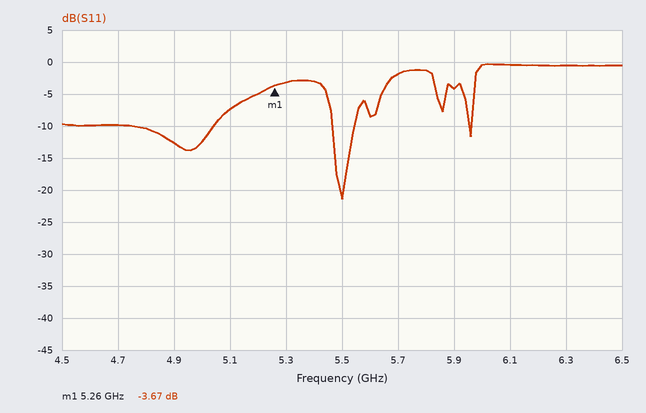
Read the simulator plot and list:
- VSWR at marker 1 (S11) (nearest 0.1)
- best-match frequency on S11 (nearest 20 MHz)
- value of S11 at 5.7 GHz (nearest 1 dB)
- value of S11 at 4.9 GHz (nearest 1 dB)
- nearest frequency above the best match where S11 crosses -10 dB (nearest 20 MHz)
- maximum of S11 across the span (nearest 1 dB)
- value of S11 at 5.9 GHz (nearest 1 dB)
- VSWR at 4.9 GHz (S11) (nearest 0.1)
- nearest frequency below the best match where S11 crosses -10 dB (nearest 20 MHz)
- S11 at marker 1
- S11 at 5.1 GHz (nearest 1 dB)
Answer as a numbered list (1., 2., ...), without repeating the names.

1. 4.8
2. 5.50 GHz
3. -2 dB
4. -13 dB
5. 5.54 GHz
6. 0 dB
7. -4 dB
8. 1.6
9. 5.46 GHz
10. -3.67 dB
11. -7 dB
